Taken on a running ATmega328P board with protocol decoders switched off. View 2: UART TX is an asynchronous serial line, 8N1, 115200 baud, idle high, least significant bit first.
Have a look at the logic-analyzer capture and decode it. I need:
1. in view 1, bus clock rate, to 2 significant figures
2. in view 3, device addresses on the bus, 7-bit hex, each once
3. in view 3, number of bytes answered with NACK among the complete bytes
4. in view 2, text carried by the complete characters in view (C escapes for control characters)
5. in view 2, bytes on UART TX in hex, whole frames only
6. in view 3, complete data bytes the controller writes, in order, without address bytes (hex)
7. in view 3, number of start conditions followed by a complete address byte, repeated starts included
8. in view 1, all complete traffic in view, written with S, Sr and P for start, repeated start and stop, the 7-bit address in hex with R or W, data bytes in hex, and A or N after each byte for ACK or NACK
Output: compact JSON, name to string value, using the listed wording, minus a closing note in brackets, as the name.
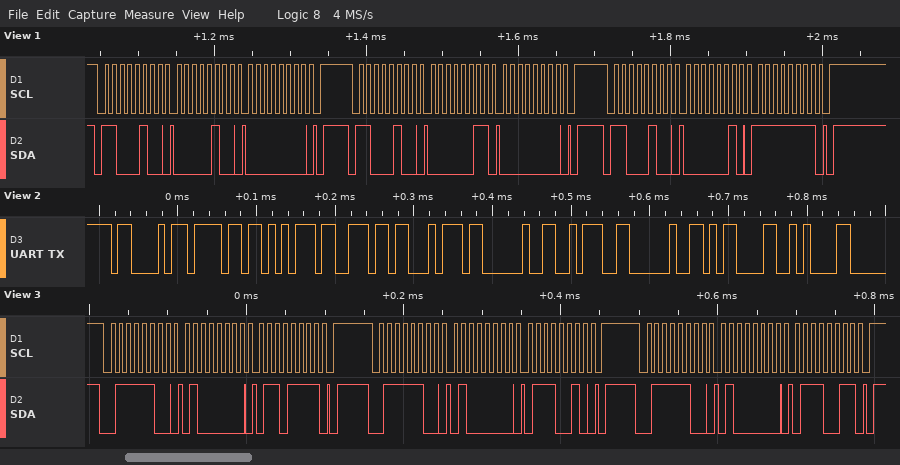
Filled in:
{"in view 1, bus clock rate, to 2 significant figures": "100 kHz", "in view 3, device addresses on the bus, 7-bit hex, each once": "0x3E", "in view 3, number of bytes answered with NACK among the complete bytes": "0", "in view 2, text carried by the complete characters in view": "\"Count : \\r\\n\"", "in view 2, bytes on UART TX in hex, whole frames only": "0x43 0x6F 0x75 0x6E 0x74 0x20 0x3A 0x20 0x0D 0x0A", "in view 3, complete data bytes the controller writes, in order, without address bytes": "40 6F 40 72 40 73", "in view 3, number of start conditions followed by a complete address byte, repeated starts included": "3", "in view 1, all complete traffic in view, written with S, Sr and P for start, repeated start and stop, the 7-bit address in hex with R or W, data bytes in hex, and A or N after each byte for ACK or NACK": "S 62W A 04 A 00 A P S 62W A 03 A 00 A P S 62W A 02 A FF A P"}
